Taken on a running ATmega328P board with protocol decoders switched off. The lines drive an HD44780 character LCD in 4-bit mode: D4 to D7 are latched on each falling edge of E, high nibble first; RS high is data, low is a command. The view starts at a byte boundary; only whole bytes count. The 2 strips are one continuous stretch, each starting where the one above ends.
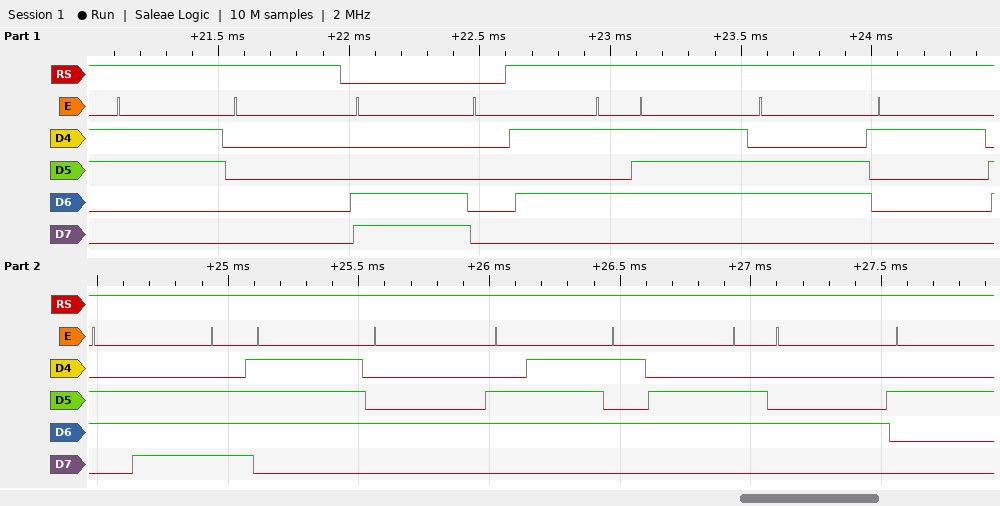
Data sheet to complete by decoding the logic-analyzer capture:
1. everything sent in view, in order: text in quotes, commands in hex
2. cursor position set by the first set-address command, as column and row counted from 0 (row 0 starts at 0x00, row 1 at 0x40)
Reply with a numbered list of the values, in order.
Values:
1. "0" 0xC0 "Wanted"
2. column 0, row 1
